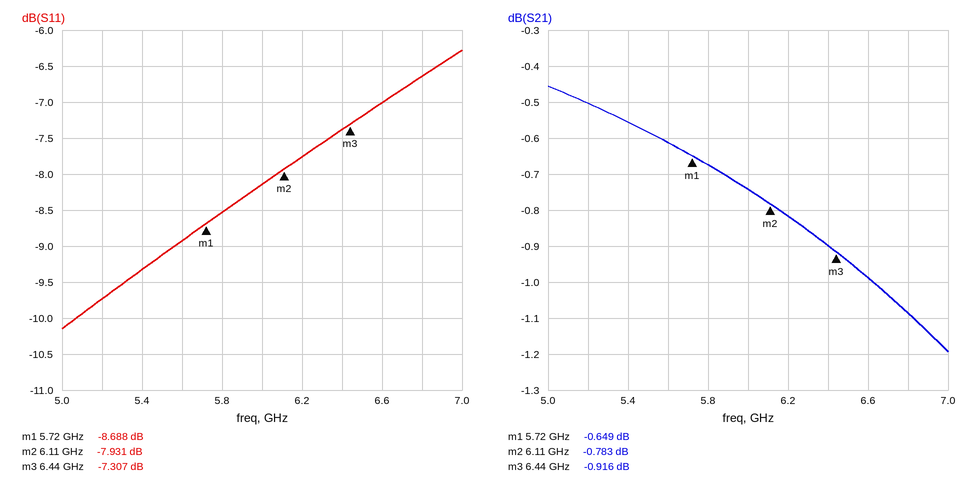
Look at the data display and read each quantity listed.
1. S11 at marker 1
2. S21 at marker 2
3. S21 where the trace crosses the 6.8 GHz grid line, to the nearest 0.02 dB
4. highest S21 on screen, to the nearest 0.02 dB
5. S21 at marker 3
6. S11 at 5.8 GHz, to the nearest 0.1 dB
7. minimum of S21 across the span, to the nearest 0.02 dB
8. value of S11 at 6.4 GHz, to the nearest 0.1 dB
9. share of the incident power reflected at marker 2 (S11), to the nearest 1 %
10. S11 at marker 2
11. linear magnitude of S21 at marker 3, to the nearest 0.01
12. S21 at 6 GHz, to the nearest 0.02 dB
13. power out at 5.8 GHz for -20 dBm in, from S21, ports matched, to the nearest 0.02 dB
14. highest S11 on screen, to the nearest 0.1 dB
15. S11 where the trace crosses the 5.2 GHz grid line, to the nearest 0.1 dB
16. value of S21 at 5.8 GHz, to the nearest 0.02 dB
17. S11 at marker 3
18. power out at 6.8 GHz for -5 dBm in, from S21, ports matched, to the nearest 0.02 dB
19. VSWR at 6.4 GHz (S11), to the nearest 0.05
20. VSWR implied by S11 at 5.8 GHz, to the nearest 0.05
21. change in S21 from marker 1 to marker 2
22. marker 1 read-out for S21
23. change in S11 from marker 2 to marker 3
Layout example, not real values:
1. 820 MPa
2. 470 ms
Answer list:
1. -8.688 dB
2. -0.783 dB
3. -1.08 dB
4. -0.46 dB
5. -0.916 dB
6. -8.5 dB
7. -1.20 dB
8. -7.4 dB
9. 16 %
10. -7.931 dB
11. 0.90
12. -0.74 dB
13. -20.68 dBm
14. -6.3 dB
15. -9.7 dB
16. -0.68 dB
17. -7.307 dB
18. -6.08 dBm
19. 2.50
20. 2.20
21. -0.134 dB
22. -0.649 dB
23. 0.624 dB
